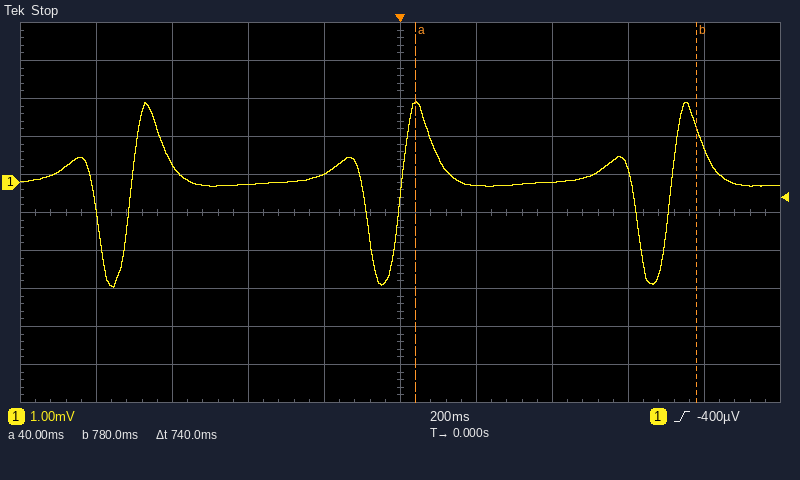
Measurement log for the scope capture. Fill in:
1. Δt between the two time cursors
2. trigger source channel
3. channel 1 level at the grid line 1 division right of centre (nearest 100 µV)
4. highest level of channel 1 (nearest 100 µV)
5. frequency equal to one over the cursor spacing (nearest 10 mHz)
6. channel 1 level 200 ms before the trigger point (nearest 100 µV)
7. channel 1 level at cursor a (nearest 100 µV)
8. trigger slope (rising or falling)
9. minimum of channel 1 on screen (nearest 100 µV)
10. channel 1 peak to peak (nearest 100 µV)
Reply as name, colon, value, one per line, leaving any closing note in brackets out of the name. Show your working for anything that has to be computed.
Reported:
Δt between the two time cursors: 740 ms
trigger source channel: channel 1
channel 1 level at the grid line 1 division right of centre: -100 µV
highest level of channel 1: 2.1 mV
frequency equal to one over the cursor spacing: 1 / 740 ms ≈ 1.35 Hz
channel 1 level 200 ms before the trigger point: 200 µV
channel 1 level at cursor a: 2.0 mV
trigger slope: rising
minimum of channel 1 on screen: -2.8 mV
channel 1 peak to peak: 2.1 mV − (-2.8 mV) = 4.9 mV
